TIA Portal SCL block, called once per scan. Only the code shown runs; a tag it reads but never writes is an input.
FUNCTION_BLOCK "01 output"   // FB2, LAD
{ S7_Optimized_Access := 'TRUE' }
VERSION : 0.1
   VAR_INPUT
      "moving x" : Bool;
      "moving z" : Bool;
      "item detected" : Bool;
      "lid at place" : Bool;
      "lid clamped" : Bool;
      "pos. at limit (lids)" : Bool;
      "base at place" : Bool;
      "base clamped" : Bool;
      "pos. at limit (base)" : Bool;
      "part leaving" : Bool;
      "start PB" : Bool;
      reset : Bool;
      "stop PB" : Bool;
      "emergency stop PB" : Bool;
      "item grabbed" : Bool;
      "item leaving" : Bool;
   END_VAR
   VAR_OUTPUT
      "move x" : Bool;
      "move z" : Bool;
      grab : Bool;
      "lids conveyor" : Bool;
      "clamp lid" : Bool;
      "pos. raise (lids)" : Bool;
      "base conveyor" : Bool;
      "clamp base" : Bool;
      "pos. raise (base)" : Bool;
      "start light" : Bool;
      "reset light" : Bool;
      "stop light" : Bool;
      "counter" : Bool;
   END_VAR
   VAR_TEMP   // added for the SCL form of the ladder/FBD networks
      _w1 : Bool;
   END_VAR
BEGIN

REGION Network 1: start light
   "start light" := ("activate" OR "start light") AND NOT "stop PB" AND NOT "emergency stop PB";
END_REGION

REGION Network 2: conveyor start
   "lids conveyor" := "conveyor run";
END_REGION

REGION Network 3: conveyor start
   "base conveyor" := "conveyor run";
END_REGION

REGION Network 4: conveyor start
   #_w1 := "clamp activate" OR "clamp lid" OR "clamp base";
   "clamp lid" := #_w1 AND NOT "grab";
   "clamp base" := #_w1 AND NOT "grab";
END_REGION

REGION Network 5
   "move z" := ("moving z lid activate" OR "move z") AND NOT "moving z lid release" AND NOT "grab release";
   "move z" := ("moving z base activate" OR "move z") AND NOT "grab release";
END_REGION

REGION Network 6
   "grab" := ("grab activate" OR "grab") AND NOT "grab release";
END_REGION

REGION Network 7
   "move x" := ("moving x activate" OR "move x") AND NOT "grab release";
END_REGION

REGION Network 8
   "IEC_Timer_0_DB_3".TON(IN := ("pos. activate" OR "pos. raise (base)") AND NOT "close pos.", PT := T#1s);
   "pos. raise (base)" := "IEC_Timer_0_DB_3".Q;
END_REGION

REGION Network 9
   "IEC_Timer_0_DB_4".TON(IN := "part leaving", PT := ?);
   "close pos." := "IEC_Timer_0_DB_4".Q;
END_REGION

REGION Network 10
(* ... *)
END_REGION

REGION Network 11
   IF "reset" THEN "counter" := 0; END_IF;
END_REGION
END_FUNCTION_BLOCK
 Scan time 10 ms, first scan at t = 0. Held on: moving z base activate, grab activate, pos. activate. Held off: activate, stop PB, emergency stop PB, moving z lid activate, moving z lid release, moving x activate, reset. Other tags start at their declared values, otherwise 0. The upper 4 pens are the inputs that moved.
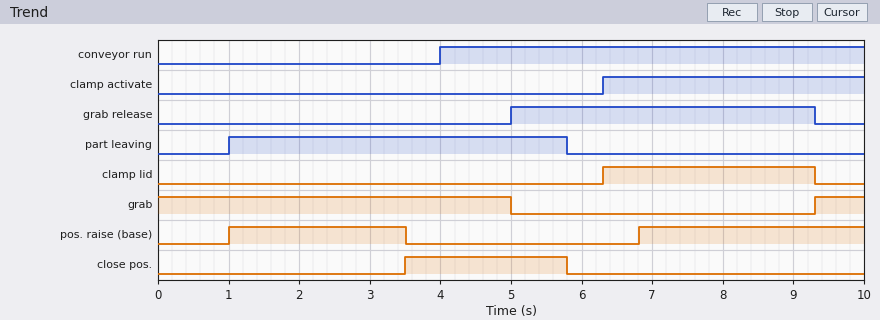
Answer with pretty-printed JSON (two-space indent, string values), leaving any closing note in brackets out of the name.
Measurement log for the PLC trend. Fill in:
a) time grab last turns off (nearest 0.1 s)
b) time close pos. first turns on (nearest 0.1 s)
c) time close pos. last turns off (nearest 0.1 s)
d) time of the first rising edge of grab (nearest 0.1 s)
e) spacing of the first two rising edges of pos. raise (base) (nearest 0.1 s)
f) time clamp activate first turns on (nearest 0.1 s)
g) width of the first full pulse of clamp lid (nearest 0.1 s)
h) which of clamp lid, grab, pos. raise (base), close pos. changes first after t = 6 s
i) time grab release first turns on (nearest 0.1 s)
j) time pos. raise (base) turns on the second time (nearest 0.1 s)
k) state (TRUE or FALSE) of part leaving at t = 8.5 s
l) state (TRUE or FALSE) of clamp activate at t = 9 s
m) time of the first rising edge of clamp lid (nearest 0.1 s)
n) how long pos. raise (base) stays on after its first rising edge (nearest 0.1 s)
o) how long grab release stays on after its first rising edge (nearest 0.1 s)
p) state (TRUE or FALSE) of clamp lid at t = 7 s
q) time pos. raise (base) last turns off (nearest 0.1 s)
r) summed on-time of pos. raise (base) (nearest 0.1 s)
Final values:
{
  "time grab last turns off": "5.0 s",
  "time close pos. first turns on": "3.5 s",
  "time close pos. last turns off": "5.8 s",
  "time of the first rising edge of grab": "9.3 s",
  "spacing of the first two rising edges of pos. raise (base)": "5.8 s",
  "time clamp activate first turns on": "6.3 s",
  "width of the first full pulse of clamp lid": "3.0 s",
  "which of clamp lid, grab, pos. raise (base), close pos. changes first after t = 6 s": "clamp lid",
  "time grab release first turns on": "5.0 s",
  "time pos. raise (base) turns on the second time": "6.8 s",
  "state (TRUE or FALSE) of part leaving at t = 8.5 s": "FALSE",
  "state (TRUE or FALSE) of clamp activate at t = 9 s": "TRUE",
  "time of the first rising edge of clamp lid": "6.3 s",
  "how long pos. raise (base) stays on after its first rising edge": "2.5 s",
  "how long grab release stays on after its first rising edge": "4.3 s",
  "state (TRUE or FALSE) of clamp lid at t = 7 s": "TRUE",
  "time pos. raise (base) last turns off": "3.5 s",
  "summed on-time of pos. raise (base)": "5.7 s"
}
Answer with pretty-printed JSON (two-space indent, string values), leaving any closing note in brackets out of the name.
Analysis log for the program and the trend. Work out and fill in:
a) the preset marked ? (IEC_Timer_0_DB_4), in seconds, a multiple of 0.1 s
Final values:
{
  "the preset marked ? (IEC_Timer_0_DB_4), in seconds, a multiple of 0.1 s": "2.5 s"
}
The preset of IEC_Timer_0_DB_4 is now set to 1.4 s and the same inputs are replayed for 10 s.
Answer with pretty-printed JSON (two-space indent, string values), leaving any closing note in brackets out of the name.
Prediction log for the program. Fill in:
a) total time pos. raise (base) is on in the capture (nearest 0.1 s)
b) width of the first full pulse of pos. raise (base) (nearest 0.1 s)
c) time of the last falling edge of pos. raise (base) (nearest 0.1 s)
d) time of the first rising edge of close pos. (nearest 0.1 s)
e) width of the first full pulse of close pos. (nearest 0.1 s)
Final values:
{
  "total time pos. raise (base) is on in the capture": "4.6 s",
  "width of the first full pulse of pos. raise (base)": "1.4 s",
  "time of the last falling edge of pos. raise (base)": "2.4 s",
  "time of the first rising edge of close pos.": "2.4 s",
  "width of the first full pulse of close pos.": "3.4 s"
}
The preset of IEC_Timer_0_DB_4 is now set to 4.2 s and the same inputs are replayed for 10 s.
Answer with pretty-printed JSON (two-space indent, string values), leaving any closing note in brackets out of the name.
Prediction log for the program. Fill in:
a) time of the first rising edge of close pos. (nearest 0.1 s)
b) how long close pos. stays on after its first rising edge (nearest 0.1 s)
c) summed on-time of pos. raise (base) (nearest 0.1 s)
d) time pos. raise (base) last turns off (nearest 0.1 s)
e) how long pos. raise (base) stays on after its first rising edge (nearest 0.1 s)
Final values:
{
  "time of the first rising edge of close pos.": "5.2 s",
  "how long close pos. stays on after its first rising edge": "0.6 s",
  "summed on-time of pos. raise (base)": "7.4 s",
  "time pos. raise (base) last turns off": "5.2 s",
  "how long pos. raise (base) stays on after its first rising edge": "4.2 s"
}
